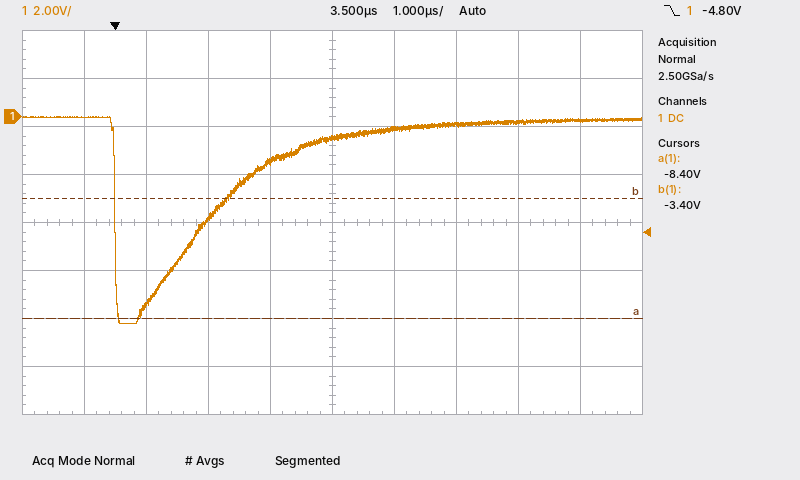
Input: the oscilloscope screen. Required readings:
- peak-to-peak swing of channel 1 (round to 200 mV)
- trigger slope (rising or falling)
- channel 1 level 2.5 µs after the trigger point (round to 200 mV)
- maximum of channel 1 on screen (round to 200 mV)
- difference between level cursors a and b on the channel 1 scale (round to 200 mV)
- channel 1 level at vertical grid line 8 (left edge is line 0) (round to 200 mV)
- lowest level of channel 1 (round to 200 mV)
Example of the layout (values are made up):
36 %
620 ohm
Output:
8.6 V
falling
-1.8 V
0.0 V
5.0 V
-200 mV
-8.6 V
